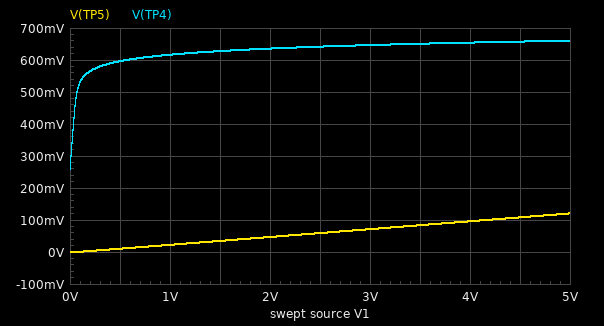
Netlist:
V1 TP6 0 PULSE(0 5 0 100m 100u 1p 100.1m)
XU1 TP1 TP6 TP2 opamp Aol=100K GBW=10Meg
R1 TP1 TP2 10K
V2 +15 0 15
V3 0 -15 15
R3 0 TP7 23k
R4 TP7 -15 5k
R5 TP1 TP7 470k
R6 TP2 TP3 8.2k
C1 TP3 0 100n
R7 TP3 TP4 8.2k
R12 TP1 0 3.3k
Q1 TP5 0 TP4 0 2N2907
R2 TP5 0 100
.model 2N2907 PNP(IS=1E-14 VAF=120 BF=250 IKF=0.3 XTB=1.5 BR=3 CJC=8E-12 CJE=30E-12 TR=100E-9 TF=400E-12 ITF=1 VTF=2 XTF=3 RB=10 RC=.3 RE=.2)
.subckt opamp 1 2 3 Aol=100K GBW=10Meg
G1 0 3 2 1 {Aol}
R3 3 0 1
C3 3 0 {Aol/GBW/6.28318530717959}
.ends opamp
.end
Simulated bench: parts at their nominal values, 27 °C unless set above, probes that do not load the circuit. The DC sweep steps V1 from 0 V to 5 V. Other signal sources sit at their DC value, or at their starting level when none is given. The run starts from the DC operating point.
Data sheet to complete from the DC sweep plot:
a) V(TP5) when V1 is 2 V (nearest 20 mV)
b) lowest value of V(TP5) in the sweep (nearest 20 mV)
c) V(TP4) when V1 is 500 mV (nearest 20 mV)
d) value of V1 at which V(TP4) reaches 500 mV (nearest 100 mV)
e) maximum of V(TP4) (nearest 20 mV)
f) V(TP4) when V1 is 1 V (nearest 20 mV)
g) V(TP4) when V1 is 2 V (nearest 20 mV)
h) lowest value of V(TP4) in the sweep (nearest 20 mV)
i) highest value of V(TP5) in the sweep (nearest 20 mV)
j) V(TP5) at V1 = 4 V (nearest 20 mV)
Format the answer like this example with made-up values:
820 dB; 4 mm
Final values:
40 mV; 0 V; 600 mV; 100 mV; 660 mV; 620 mV; 640 mV; 260 mV; 120 mV; 100 mV
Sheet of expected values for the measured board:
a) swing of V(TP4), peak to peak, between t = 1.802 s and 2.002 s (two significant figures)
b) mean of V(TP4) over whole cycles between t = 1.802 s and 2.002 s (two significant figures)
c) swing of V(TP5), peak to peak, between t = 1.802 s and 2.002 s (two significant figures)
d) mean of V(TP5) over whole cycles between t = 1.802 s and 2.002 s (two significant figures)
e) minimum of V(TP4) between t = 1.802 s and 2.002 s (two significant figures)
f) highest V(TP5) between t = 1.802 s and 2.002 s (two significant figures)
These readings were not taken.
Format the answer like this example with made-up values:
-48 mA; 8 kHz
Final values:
120 mV; 630 mV; 120 mV; 59 mV; 540 mV; 120 mV
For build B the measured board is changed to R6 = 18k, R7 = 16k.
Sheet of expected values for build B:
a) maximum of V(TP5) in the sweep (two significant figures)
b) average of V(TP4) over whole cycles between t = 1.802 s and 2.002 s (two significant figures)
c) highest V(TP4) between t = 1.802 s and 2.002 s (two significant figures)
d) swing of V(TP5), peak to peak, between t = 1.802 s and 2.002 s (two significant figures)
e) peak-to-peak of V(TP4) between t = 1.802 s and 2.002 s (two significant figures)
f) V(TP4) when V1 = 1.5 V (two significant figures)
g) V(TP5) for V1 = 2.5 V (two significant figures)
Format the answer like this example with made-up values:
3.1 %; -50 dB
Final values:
58 mV; 620 mV; 640 mV; 56 mV; 94 mV; 610 mV; 29 mV
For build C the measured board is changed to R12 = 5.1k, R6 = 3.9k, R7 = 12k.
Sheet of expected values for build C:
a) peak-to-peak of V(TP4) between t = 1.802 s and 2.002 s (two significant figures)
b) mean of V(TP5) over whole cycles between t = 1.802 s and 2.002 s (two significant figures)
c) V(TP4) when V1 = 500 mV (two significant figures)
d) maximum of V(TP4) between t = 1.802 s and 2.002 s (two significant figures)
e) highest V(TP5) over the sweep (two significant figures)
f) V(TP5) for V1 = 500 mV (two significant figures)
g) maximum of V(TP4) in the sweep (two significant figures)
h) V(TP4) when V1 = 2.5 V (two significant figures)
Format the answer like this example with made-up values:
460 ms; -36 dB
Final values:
170 mV; 44 mV; 590 mV; 650 mV; 91 mV; 7.3 mV; 650 mV; 630 mV
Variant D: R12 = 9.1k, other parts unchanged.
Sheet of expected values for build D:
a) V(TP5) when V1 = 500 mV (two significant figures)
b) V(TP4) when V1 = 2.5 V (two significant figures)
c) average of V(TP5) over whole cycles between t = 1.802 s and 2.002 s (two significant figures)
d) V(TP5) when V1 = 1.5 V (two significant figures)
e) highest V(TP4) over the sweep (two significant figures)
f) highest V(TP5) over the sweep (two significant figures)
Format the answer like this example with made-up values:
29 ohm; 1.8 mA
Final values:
4.5 mV; 620 mV; 30 mV; 17 mV; 640 mV; 62 mV
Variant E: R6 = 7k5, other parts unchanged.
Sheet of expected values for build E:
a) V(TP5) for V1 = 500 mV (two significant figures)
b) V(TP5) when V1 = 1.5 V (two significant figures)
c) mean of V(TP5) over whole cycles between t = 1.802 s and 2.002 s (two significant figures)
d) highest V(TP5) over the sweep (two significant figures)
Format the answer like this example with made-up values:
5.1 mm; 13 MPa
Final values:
11 mV; 36 mV; 62 mV; 130 mV
